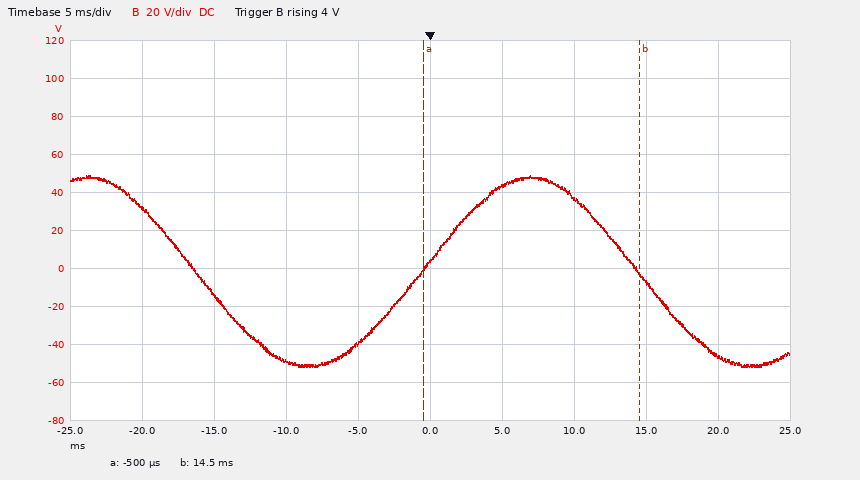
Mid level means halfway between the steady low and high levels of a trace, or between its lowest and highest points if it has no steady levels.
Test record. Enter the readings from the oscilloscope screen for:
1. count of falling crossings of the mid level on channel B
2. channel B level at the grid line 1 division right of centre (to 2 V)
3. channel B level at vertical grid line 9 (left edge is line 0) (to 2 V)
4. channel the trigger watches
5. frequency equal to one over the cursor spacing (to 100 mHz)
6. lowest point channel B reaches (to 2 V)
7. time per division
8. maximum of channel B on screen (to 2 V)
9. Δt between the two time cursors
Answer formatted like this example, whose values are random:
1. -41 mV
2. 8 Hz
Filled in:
1. 2
2. 44 V
3. -46 V
4. channel B
5. 66.7 Hz
6. -52 V
7. 5 ms
8. 48 V
9. 15.0 ms
